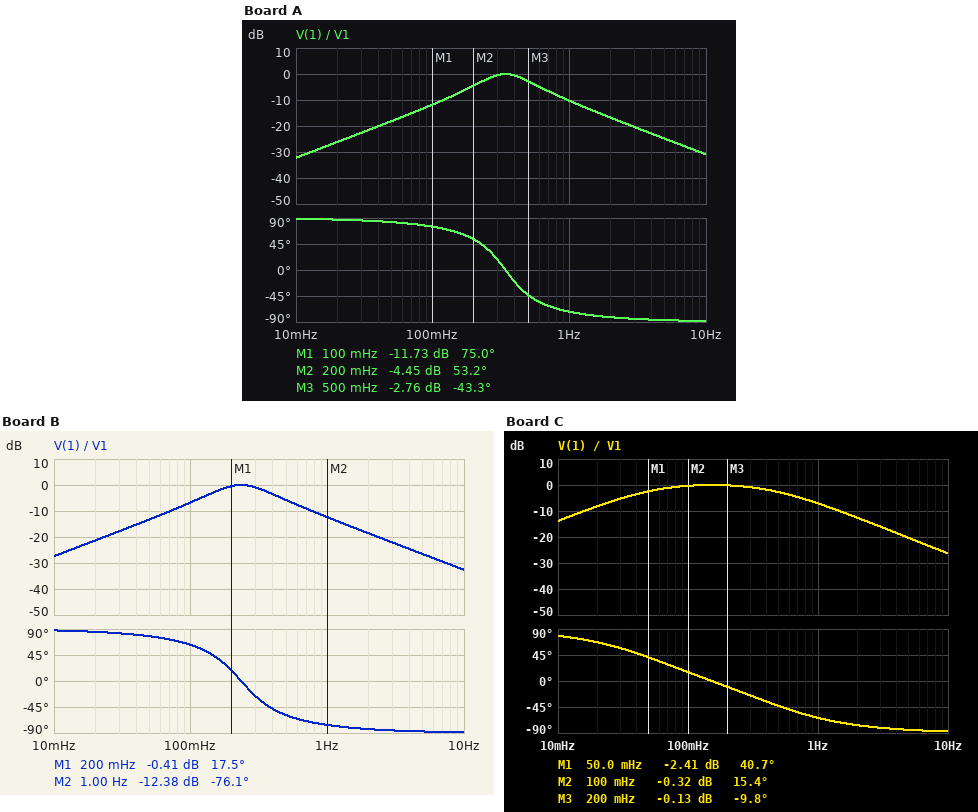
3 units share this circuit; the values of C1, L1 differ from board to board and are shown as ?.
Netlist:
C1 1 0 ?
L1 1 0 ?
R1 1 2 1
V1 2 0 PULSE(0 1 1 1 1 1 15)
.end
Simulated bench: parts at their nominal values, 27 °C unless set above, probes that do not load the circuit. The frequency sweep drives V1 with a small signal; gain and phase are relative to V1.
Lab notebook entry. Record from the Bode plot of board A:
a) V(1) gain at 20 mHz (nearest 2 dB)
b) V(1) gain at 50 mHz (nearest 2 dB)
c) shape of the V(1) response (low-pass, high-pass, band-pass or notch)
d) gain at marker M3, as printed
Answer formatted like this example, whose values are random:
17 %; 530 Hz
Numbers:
-26 dB; -18 dB; band-pass; -2.76 dB
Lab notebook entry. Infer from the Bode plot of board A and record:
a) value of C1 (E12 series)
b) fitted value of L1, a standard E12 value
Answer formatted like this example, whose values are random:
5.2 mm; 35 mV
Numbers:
560 mF; 390 mH
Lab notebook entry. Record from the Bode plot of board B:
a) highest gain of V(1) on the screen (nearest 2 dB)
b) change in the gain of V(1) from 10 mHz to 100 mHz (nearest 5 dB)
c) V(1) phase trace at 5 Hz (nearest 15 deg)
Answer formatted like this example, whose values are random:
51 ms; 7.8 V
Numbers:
0 dB; 20 dB; -90 deg
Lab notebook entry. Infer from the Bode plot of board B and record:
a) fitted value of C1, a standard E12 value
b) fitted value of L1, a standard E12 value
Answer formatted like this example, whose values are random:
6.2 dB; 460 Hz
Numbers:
680 mF; 680 mH
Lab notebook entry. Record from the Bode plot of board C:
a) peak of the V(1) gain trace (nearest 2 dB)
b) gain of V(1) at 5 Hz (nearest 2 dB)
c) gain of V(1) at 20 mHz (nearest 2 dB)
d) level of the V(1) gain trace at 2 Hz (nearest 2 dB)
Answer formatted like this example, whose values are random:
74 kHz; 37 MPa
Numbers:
0 dB; -20 dB; -8 dB; -12 dB
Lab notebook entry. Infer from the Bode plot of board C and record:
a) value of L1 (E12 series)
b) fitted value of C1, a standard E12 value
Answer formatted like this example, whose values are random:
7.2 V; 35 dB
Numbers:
3.3 H; 330 mF
